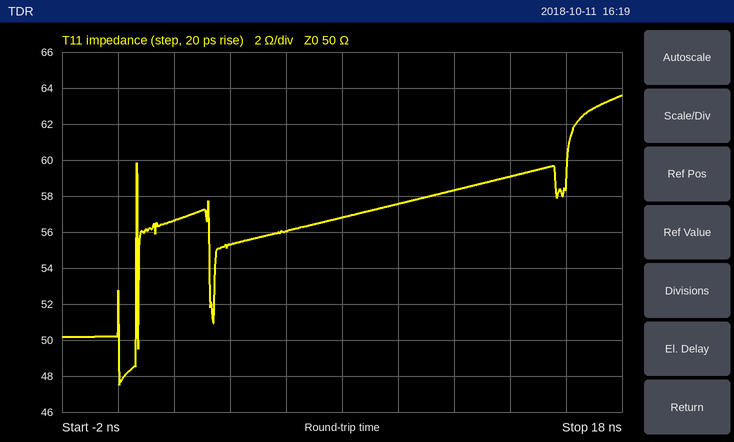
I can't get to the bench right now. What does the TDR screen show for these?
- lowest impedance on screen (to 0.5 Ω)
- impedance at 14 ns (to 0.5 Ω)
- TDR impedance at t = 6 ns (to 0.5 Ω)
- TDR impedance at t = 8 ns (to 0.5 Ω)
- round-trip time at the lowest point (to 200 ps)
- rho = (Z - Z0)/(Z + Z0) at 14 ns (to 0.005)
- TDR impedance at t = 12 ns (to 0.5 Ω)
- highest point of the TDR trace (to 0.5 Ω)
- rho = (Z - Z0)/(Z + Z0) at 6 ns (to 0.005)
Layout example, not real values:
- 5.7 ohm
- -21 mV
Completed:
- 47.5 Ω
- 59.0 Ω
- 56.0 Ω
- 57.0 Ω
- 0.0 ns
- +0.085
- 58.5 Ω
- 63.5 Ω
- +0.055
